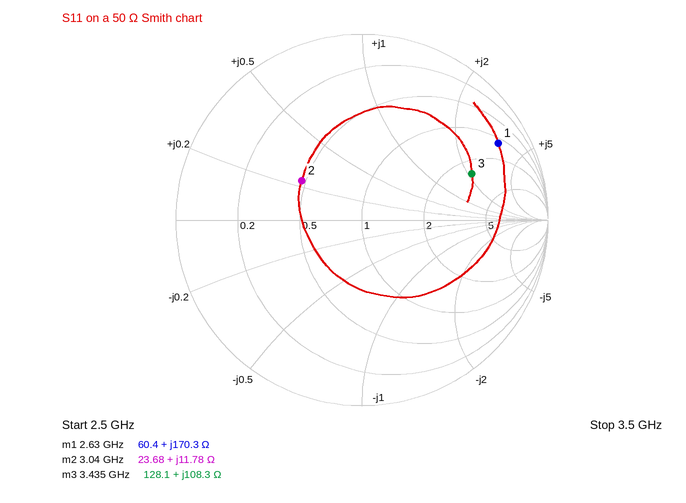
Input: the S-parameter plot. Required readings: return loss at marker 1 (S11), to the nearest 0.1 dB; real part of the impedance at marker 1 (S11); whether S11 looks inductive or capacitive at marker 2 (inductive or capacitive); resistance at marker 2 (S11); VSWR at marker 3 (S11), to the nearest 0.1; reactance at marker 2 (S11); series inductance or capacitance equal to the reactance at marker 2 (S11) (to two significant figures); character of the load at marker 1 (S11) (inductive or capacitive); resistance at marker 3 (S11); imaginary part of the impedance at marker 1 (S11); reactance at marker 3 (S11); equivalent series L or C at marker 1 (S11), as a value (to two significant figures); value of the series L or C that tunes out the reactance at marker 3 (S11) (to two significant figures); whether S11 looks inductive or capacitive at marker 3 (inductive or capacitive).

1.5 dB
60.4 Ω
inductive
23.68 Ω
4.6
+11.78 Ω
620 pH
inductive
128.1 Ω
+170.3 Ω
+108.3 Ω
10 nH
430 fF
inductive
